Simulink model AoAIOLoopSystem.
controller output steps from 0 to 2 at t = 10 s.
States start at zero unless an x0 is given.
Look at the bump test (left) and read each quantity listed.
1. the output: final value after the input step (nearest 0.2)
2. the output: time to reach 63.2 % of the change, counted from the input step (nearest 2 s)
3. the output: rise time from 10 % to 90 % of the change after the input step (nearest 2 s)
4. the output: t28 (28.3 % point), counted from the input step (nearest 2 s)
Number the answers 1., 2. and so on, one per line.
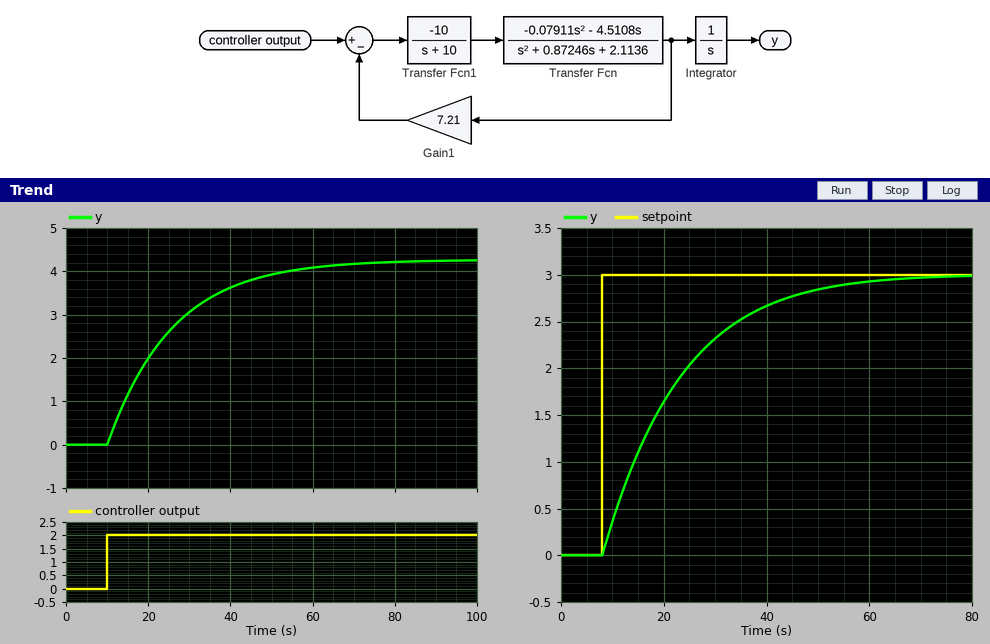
1. 4.2
2. 16 s
3. 34 s
4. 6 s
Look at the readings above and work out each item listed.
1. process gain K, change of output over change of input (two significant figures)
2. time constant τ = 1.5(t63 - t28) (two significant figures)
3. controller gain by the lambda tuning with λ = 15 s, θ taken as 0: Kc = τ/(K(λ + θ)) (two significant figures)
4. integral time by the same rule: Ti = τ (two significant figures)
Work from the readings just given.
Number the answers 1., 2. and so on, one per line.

1. 2.1
2. 15 s
3. 0.48
4. 15 s
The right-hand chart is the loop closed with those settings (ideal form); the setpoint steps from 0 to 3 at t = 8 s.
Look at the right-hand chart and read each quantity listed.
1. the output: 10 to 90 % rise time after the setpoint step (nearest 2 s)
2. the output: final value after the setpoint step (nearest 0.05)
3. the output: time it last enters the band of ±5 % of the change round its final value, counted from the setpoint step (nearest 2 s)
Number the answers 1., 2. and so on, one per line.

1. 32 s
2. 3.00
3. 42 s
